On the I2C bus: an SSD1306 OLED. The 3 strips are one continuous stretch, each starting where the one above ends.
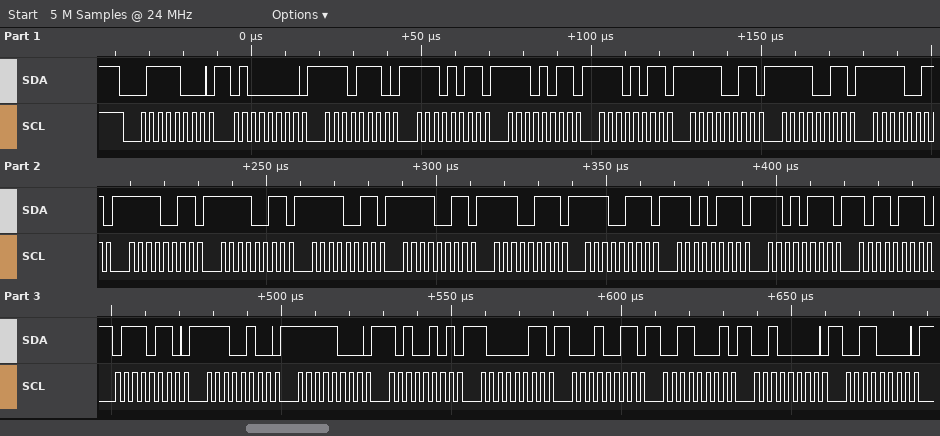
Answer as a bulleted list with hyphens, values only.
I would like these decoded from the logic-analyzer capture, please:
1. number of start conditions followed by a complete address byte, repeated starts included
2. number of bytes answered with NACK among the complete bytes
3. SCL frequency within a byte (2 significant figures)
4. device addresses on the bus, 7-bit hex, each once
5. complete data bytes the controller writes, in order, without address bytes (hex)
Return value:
- 1
- 0
- 400 kHz
- 0x3C
- 40 EE EB EB EB F3 F3 F3 F3 F3 F3 F3 E7 E7 D7 D7 B7 76 E4 F8 A5 83 13 31 20 30
